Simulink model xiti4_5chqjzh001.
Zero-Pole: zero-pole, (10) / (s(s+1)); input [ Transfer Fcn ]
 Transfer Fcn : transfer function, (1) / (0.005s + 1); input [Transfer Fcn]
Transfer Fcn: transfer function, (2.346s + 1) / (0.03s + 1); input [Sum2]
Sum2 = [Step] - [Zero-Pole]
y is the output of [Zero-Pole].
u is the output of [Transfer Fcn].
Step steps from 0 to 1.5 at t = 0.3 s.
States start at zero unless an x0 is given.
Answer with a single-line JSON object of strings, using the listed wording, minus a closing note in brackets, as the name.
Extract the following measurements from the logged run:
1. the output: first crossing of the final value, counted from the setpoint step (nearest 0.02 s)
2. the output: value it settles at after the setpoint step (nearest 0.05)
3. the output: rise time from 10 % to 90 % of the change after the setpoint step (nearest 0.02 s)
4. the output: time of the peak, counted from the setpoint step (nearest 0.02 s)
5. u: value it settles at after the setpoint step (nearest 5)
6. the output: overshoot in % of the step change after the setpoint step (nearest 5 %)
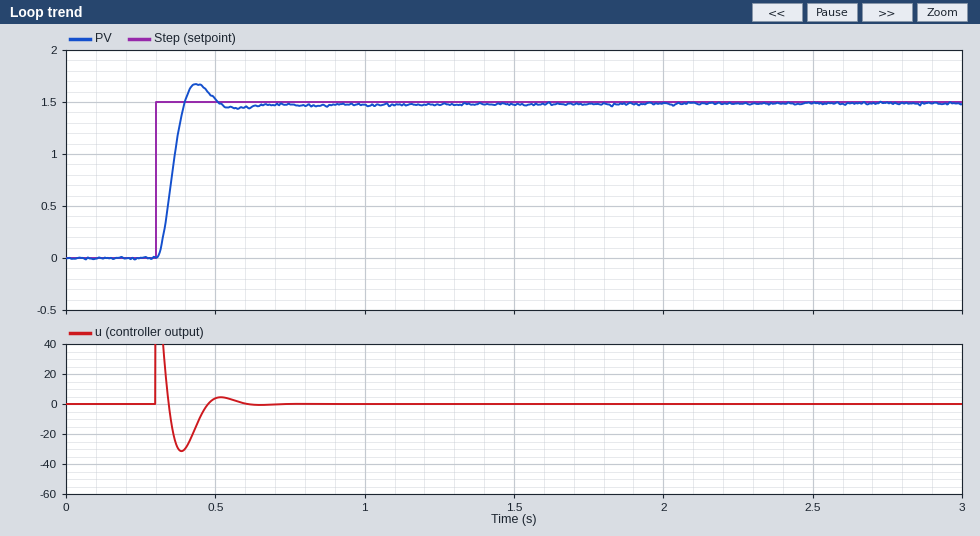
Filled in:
{"the output: first crossing of the final value, counted from the setpoint step": "0.10 s", "the output: value it settles at after the setpoint step": "1.50", "the output: rise time from 10 % to 90 % of the change after the setpoint step": "0.06 s", "the output: time of the peak, counted from the setpoint step": "0.14 s", "u: value it settles at after the setpoint step": "0", "the output: overshoot in % of the step change after the setpoint step": "10 %"}
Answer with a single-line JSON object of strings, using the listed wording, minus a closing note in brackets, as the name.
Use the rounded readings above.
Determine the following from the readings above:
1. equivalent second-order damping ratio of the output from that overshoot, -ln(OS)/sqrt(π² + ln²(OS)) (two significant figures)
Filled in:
{"equivalent second-order damping ratio of the output from that overshoot, -ln(OS)/sqrt(π² + ln²(OS))": "0.59"}
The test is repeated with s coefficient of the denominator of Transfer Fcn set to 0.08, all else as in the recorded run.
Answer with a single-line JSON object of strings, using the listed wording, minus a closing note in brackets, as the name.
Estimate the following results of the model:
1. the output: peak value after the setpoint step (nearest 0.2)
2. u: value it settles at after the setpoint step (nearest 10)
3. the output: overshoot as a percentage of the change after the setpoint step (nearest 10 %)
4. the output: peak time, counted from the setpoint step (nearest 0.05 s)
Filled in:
{"the output: peak value after the setpoint step": "2.0", "u: value it settles at after the setpoint step": "0", "the output: overshoot as a percentage of the change after the setpoint step": "30 %", "the output: peak time, counted from the setpoint step": "0.20 s"}
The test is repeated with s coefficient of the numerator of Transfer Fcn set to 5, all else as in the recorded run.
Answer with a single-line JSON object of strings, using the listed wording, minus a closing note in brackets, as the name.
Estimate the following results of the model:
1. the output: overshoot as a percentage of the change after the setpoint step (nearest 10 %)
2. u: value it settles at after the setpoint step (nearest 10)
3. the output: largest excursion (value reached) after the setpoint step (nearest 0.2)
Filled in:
{"the output: overshoot as a percentage of the change after the setpoint step": "30 %", "u: value it settles at after the setpoint step": "0", "the output: largest excursion (value reached) after the setpoint step": "2.0"}
